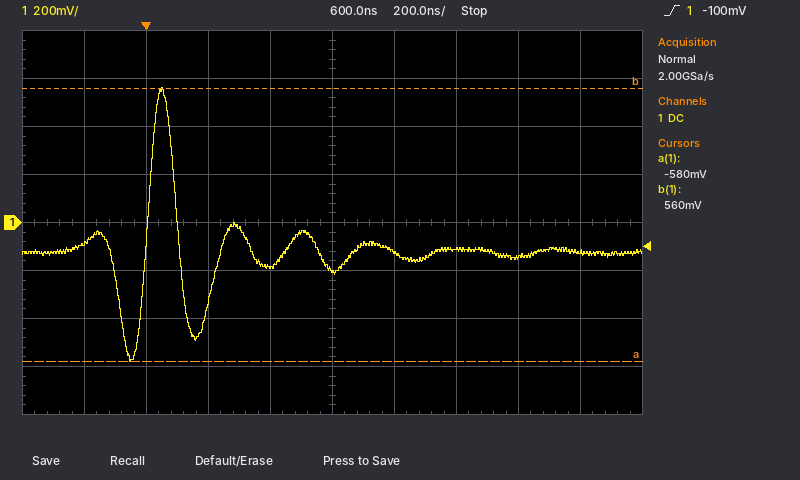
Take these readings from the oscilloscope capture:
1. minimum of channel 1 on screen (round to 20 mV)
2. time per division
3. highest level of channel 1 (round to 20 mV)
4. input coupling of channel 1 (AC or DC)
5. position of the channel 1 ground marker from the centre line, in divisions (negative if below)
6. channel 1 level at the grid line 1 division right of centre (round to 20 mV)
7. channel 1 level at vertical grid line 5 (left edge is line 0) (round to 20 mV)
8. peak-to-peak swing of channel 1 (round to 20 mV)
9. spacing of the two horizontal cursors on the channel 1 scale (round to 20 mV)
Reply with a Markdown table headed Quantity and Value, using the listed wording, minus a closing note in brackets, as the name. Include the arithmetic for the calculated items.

| Quantity | Value |
|---|---|
| minimum of channel 1 on screen | -580 mV |
| time per division | 200 ns |
| highest level of channel 1 | 560 mV |
| input coupling of channel 1 | DC |
| position of the channel 1 ground marker from the centre line, in divisions | 0.0 div |
| channel 1 level at the grid line 1 division right of centre | -120 mV |
| channel 1 level at vertical grid line 5 (left edge is line 0) | -200 mV |
| peak-to-peak swing of channel 1 | 560 mV − (-580 mV) = 1.14 V |
| spacing of the two horizontal cursors on the channel 1 scale | 1.14 V |
